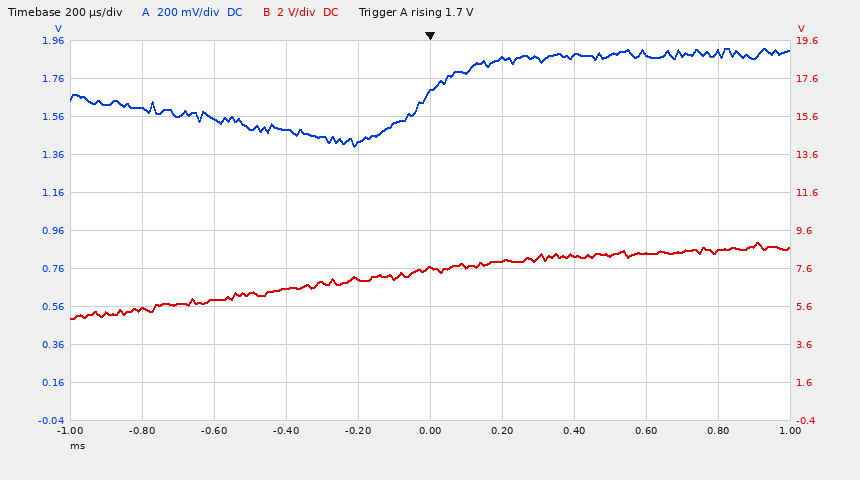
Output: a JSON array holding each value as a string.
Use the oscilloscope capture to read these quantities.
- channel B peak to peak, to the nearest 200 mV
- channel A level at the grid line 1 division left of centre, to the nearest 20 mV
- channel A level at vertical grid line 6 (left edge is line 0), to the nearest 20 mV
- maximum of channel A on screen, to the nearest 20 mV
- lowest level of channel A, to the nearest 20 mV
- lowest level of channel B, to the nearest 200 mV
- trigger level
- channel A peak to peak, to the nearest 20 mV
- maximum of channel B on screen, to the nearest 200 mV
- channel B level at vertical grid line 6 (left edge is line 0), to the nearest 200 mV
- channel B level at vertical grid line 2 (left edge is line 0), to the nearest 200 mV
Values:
["4.0 V", "1.42 V", "1.86 V", "1.92 V", "1.40 V", "5.0 V", "1.7 V", "520 mV", "9.0 V", "8.0 V", "6.0 V"]
